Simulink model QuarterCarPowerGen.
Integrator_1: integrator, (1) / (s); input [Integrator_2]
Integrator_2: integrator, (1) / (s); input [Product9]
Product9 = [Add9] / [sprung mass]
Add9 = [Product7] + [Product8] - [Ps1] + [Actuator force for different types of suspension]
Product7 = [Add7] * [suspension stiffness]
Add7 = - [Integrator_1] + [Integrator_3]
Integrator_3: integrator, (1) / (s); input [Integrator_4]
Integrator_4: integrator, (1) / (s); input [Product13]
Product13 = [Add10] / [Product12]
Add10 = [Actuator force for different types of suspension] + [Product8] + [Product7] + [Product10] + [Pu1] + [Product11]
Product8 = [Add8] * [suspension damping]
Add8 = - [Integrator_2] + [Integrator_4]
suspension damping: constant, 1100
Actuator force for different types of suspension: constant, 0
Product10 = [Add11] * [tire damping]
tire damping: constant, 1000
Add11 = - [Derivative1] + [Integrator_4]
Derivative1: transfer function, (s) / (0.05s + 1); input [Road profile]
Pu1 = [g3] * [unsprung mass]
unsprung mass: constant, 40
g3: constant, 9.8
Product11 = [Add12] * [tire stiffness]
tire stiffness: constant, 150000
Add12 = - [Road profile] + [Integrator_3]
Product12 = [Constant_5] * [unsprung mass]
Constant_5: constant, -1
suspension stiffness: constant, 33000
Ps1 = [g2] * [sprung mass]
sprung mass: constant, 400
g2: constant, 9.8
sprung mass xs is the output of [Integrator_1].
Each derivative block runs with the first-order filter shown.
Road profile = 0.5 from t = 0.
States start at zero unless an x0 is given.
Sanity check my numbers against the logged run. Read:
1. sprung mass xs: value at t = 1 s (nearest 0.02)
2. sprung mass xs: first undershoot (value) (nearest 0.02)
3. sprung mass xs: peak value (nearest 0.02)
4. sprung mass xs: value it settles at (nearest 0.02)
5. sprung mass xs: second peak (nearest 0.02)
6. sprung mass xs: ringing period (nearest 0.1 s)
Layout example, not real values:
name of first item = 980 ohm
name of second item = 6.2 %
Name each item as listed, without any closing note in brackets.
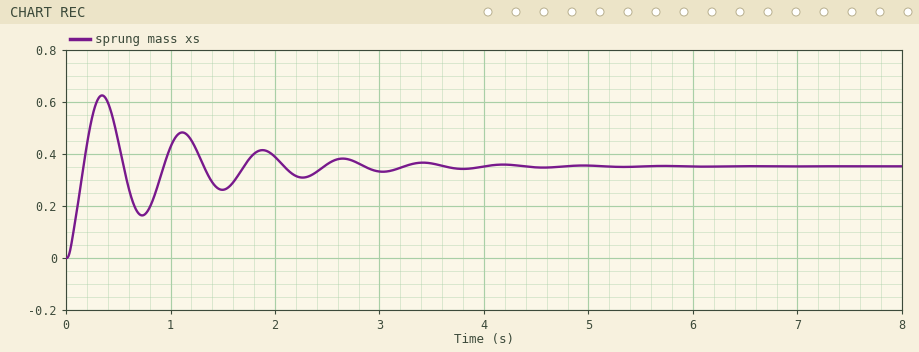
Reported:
sprung mass xs: value at t = 1 s = 0.42
sprung mass xs: first undershoot (value) = 0.16
sprung mass xs: peak value = 0.62
sprung mass xs: value it settles at = 0.36
sprung mass xs: second peak = 0.48
sprung mass xs: ringing period = 0.8 s
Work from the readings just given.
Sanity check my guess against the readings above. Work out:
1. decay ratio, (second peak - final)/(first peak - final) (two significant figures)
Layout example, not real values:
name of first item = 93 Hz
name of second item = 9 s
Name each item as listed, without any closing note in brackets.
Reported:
decay ratio, (second peak - final)/(first peak - final) = 0.46
